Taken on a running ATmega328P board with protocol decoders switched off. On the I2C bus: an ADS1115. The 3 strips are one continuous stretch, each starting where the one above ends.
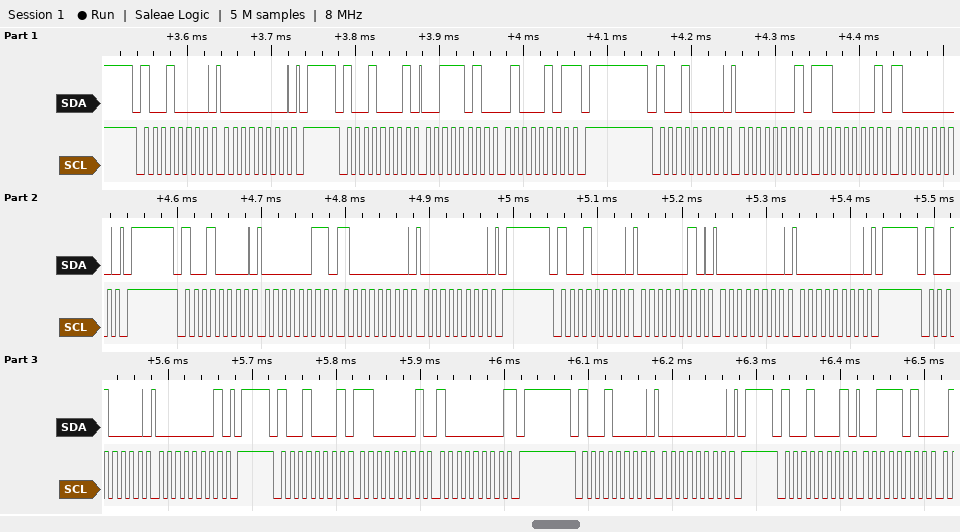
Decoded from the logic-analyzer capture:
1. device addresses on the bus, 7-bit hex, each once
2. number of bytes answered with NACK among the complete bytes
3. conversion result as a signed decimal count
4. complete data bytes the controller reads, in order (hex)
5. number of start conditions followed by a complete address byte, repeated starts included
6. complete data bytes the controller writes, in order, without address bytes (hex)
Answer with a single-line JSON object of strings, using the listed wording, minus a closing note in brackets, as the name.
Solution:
{"device addresses on the bus, 7-bit hex, each once": "0x48", "number of bytes answered with NACK among the complete bytes": "2", "conversion result as a signed decimal count": "14917", "complete data bytes the controller reads, in order": "3A 45 C1 80 3A", "number of start conditions followed by a complete address byte, repeated starts included": "9", "complete data bytes the controller writes, in order, without address bytes": "00 01 C1 80 03 80 00 02 00 00 01 00"}
